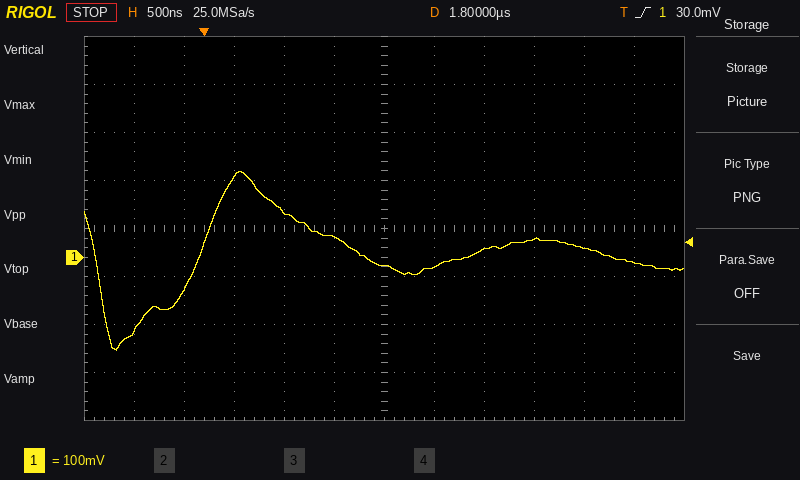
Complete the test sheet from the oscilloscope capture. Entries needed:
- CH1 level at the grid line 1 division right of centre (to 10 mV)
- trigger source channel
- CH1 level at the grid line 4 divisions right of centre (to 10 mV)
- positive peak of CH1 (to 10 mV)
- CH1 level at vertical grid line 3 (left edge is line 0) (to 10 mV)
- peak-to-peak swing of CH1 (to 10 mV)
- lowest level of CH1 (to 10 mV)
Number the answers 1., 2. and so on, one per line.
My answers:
1. -20 mV
2. CH1
3. 20 mV
4. 180 mV
5. 170 mV
6. 370 mV
7. -190 mV
